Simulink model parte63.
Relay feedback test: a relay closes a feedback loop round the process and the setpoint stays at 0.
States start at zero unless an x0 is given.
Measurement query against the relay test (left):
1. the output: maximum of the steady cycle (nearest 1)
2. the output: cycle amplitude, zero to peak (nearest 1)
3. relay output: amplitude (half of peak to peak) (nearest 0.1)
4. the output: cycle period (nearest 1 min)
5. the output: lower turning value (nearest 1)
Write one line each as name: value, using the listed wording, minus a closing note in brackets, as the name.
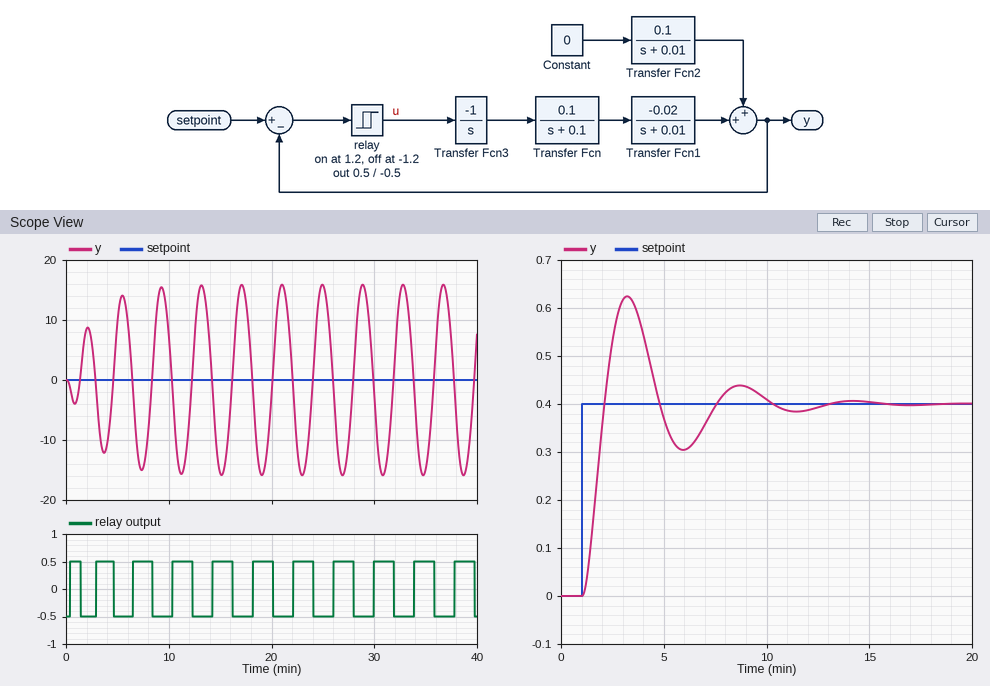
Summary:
the output: maximum of the steady cycle: 16
the output: cycle amplitude, zero to peak: 16
relay output: amplitude (half of peak to peak): 0.5
the output: cycle period: 4 min
the output: lower turning value: -16
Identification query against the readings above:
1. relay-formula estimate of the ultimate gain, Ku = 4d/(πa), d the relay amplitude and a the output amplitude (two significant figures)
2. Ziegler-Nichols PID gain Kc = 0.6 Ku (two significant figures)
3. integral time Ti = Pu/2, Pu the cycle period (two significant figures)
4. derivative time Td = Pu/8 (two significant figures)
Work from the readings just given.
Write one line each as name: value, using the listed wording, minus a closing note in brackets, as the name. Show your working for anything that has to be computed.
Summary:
relay-formula estimate of the ultimate gain, Ku = 4d/(πa), d the relay amplitude and a the output amplitude: 4 × 0.5 / (π × 16) = 0.040
Ziegler-Nichols PID gain Kc = 0.6 Ku: 0.6 × 0.04 = 0.024
integral time Ti = Pu/2, Pu the cycle period: 4 / 2 = 2.0 min
derivative time Td = Pu/8: 4 / 8 = 0.50 min
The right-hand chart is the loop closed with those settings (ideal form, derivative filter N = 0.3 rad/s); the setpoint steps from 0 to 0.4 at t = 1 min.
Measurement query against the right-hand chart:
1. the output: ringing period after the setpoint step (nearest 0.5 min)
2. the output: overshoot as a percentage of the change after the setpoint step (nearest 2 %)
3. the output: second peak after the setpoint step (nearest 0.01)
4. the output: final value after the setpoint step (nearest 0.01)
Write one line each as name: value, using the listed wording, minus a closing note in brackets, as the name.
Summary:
the output: ringing period after the setpoint step: 5.5 min
the output: overshoot as a percentage of the change after the setpoint step: 56 %
the output: second peak after the setpoint step: 0.44
the output: final value after the setpoint step: 0.40
